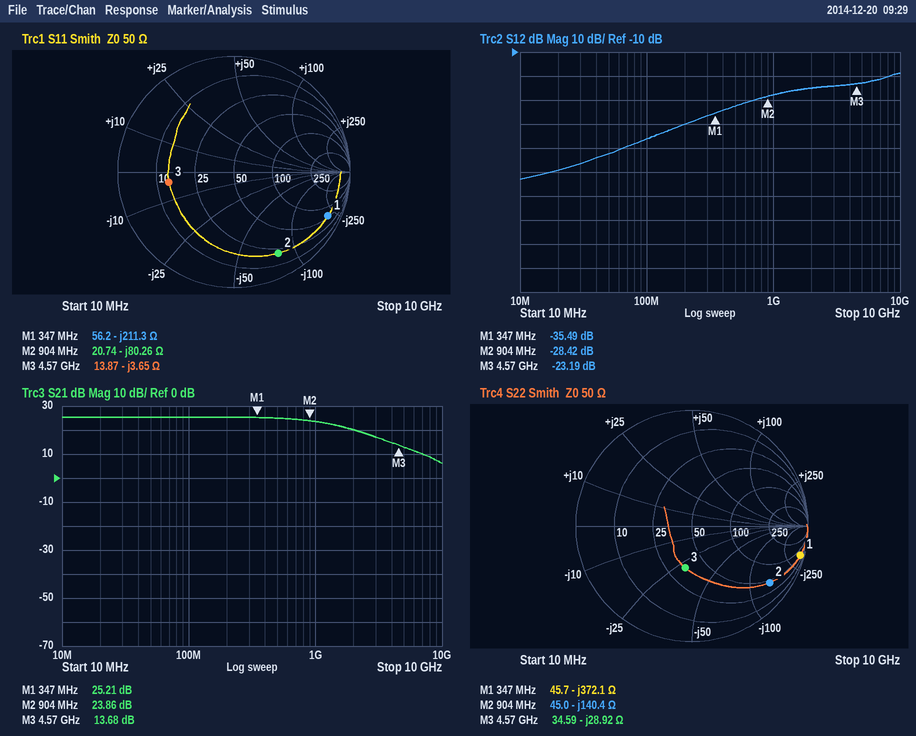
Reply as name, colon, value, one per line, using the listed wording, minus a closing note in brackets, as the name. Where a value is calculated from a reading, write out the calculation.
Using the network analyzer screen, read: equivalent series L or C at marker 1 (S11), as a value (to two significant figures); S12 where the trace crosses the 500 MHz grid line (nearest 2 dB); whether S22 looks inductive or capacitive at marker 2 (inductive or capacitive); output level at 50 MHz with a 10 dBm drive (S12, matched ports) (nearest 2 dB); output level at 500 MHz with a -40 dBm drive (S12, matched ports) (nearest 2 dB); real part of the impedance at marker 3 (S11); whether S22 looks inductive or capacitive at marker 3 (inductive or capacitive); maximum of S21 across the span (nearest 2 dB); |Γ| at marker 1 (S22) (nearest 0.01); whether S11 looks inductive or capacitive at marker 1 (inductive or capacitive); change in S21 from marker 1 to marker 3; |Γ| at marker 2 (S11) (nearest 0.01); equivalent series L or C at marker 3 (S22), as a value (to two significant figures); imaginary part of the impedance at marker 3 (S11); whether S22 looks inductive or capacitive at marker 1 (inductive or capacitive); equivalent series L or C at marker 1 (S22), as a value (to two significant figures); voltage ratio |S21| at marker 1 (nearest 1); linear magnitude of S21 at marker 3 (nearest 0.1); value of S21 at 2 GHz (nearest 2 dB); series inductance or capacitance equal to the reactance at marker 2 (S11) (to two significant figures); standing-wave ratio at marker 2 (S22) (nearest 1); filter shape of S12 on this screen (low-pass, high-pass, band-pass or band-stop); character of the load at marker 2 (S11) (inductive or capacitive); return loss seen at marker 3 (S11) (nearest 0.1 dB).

equivalent series L or C at marker 1 (S11), as a value: C = 1/(2π × 347 MHz × 211.3 Ω) ≈ 2.2 pF
S12 where the trace crosses the 500 MHz grid line: -32 dB
whether S22 looks inductive or capacitive at marker 2: capacitive
output level at 50 MHz with a 10 dBm drive (S12, matched ports): 10 dBm + (-52 dB) = -42 dBm
output level at 500 MHz with a -40 dBm drive (S12, matched ports): -40 dBm + (-32 dB) = -72 dBm
real part of the impedance at marker 3: 13.87 Ω
whether S22 looks inductive or capacitive at marker 3: capacitive
maximum of S21 across the span: 26 dB
|Γ| at marker 1 (S22): 0.97
whether S11 looks inductive or capacitive at marker 1: capacitive
change in S21 from marker 1 to marker 3: 13.68 − (25.21) = -11.53 dB
|Γ| at marker 2 (S11): 0.80
equivalent series L or C at marker 3 (S22), as a value: C = 1/(2π × 4.57 GHz × 28.92 Ω) ≈ 1.2 pF
imaginary part of the impedance at marker 3: -3.65 Ω
whether S22 looks inductive or capacitive at marker 1: capacitive
equivalent series L or C at marker 1 (S22), as a value: C = 1/(2π × 347 MHz × 372.1 Ω) ≈ 1.2 pF
voltage ratio |S21| at marker 1: 10^(25.21/20) ≈ 18
linear magnitude of S21 at marker 3: 10^(13.68/20) ≈ 4.8
value of S21 at 2 GHz: 20 dB
series inductance or capacitance equal to the reactance at marker 2 (S11): C = 1/(2π × 904 MHz × 80.26 Ω) ≈ 2.2 pF
standing-wave ratio at marker 2 (S22): 11
filter shape of S12 on this screen: high-pass
character of the load at marker 2 (S11): capacitive
return loss seen at marker 3 (S11): 4.9 dB
